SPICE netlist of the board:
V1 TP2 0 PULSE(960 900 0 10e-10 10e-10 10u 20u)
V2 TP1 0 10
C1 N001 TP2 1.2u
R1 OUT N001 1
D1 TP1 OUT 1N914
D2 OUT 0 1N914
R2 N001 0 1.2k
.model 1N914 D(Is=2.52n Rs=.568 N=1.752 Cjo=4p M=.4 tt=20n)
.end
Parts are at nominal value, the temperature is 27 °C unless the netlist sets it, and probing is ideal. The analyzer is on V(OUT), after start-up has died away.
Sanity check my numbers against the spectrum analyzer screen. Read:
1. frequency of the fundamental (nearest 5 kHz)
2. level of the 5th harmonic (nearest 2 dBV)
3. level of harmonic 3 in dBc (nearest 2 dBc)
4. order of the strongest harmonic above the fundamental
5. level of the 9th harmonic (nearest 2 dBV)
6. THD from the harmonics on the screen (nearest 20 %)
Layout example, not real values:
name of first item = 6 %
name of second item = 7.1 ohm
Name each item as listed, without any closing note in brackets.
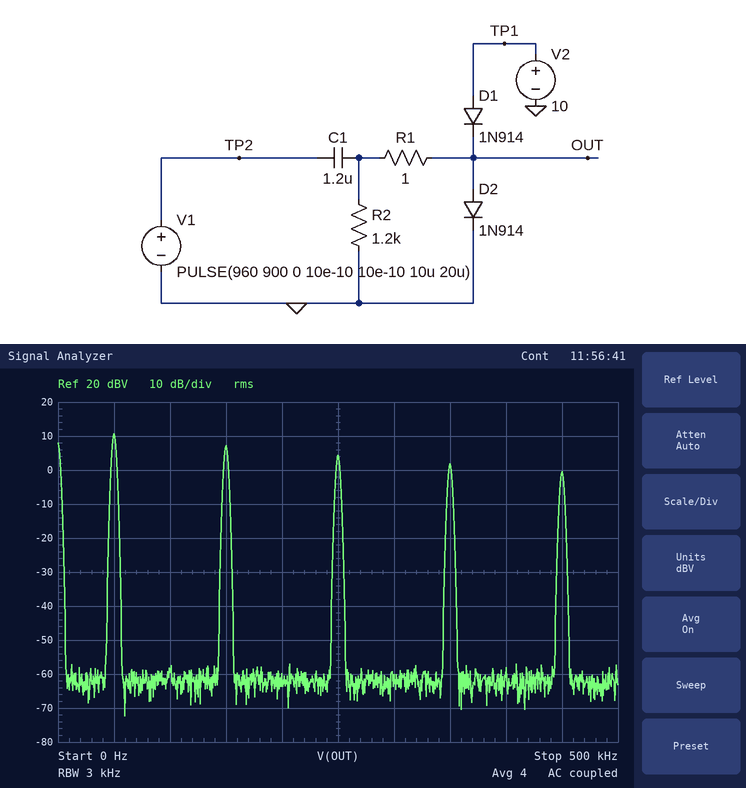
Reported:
frequency of the fundamental = 50 kHz
level of the 5th harmonic = 4 dBV
level of harmonic 3 in dBc = -4 dBc
order of the strongest harmonic above the fundamental = 3
level of the 9th harmonic = 0 dBV
THD from the harmonics on the screen = 100 %
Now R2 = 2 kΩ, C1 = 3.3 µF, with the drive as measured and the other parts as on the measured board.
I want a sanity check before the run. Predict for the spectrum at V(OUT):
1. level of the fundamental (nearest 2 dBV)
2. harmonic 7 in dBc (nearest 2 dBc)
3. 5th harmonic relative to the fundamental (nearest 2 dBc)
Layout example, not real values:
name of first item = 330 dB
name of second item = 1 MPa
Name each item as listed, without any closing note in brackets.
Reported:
level of the fundamental = 16 dBV
harmonic 7 in dBc = -14 dBc
5th harmonic relative to the fundamental = -12 dBc
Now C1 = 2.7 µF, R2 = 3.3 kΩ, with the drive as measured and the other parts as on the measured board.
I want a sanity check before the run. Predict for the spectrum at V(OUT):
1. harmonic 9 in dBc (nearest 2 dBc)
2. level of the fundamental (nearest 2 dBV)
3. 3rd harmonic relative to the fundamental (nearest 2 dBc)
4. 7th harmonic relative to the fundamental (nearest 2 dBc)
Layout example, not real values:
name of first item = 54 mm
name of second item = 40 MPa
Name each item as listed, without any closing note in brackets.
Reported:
harmonic 9 in dBc = -16 dBc
level of the fundamental = 16 dBV
3rd harmonic relative to the fundamental = -6 dBc
7th harmonic relative to the fundamental = -14 dBc
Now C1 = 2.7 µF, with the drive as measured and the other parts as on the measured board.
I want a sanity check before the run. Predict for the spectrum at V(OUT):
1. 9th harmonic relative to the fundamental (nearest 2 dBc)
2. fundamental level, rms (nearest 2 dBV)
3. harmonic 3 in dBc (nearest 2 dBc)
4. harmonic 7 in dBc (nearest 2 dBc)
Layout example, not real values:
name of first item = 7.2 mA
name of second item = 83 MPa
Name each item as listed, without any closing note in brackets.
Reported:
9th harmonic relative to the fundamental = -16 dBc
fundamental level, rms = 16 dBV
harmonic 3 in dBc = -6 dBc
harmonic 7 in dBc = -14 dBc
